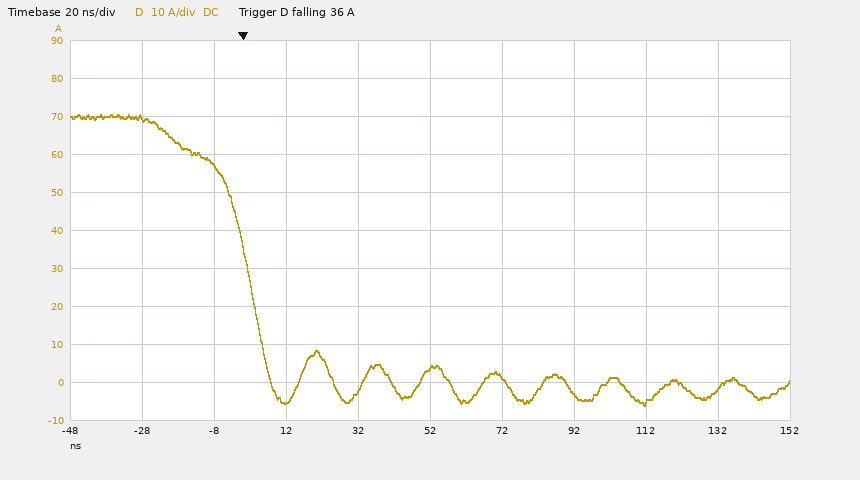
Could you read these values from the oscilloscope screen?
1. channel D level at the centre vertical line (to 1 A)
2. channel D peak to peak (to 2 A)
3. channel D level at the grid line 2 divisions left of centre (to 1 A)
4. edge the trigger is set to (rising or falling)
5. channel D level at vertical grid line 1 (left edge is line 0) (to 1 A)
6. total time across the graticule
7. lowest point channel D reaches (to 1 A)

4 A
76 A
-5 A
falling
70 A
200 ns
-6 A
